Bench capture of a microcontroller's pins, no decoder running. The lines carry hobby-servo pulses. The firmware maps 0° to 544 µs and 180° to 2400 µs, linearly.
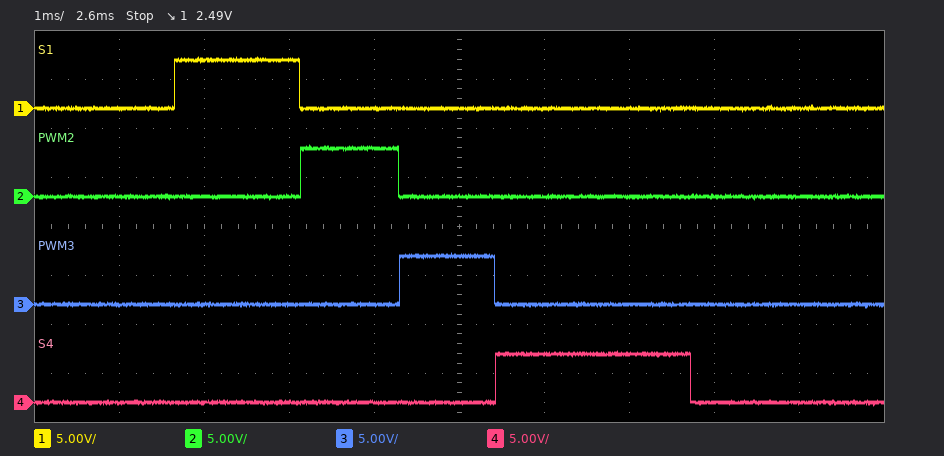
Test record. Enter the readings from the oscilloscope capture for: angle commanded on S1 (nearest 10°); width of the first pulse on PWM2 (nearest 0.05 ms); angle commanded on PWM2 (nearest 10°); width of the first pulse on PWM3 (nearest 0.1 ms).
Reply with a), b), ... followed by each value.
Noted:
a) 90°
b) 1.15 ms
c) 60°
d) 1.1 ms
